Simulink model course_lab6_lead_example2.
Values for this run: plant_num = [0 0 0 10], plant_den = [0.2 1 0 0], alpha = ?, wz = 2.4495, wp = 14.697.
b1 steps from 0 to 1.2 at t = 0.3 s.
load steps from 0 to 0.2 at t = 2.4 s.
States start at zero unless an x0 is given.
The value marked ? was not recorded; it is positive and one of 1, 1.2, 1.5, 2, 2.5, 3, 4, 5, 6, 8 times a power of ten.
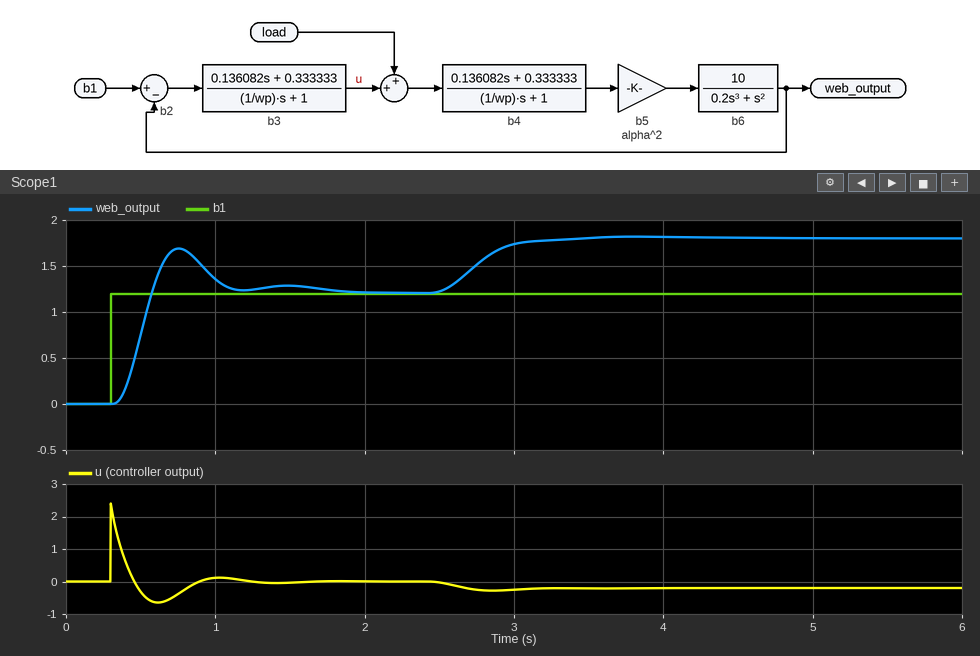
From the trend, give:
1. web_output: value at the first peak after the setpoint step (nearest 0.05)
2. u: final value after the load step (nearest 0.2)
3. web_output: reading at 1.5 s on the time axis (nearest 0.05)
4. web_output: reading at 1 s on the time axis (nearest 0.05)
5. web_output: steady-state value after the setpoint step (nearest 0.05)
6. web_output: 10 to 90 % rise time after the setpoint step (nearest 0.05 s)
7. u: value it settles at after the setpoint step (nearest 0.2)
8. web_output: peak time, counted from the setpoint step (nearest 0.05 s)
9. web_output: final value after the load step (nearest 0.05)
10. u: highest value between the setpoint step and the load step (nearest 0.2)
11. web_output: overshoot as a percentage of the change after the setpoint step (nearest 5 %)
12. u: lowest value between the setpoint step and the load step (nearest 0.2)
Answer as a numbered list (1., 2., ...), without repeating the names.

1. 1.70
2. -0.2
3. 1.30
4. 1.35
5. 1.20
6. 0.15 s
7. 0.0
8. 0.45 s
9. 1.80
10. 2.4
11. 40 %
12. -0.6
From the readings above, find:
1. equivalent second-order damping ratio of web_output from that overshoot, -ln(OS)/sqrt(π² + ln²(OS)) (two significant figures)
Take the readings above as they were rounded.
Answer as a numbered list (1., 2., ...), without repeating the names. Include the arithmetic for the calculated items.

1. ln(0.4) = -0.916; 0.916 / sqrt(9.870 + 0.840) = 0.28
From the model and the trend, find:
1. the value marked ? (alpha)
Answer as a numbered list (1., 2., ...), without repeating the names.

1. 3
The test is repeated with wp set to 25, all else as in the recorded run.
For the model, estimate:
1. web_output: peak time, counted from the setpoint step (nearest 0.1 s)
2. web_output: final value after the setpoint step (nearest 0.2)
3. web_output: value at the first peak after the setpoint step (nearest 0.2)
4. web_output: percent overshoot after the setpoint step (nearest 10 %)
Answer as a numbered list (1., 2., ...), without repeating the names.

1. 0.4 s
2. 1.2
3. 1.4
4. 20 %
